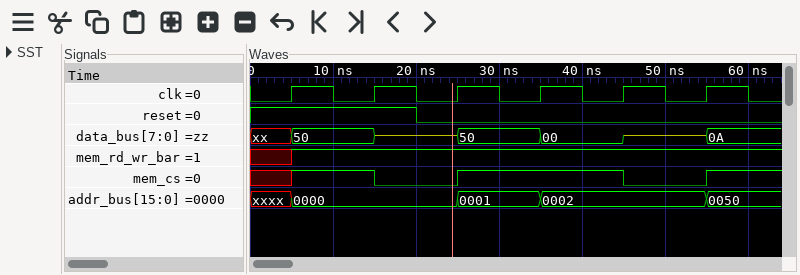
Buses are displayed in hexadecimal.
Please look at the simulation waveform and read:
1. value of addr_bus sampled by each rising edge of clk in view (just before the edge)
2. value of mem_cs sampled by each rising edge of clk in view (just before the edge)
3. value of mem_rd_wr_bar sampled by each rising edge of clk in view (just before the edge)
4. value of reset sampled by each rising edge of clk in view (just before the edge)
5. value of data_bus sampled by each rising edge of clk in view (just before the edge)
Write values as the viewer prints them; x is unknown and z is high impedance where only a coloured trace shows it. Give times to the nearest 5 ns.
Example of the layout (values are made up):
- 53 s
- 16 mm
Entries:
- xxxx, 0000, 0000, 0001, 0002, 0002
- x 1 0 1 1 0
- x 1 1 1 1 1
- 1 1 0 0 0 0
- xx, 50, z, 50, 00, z
